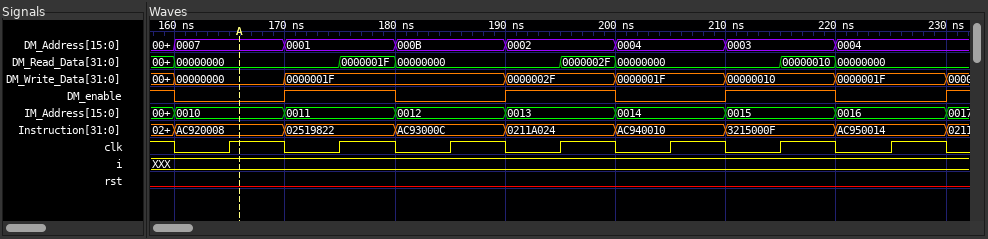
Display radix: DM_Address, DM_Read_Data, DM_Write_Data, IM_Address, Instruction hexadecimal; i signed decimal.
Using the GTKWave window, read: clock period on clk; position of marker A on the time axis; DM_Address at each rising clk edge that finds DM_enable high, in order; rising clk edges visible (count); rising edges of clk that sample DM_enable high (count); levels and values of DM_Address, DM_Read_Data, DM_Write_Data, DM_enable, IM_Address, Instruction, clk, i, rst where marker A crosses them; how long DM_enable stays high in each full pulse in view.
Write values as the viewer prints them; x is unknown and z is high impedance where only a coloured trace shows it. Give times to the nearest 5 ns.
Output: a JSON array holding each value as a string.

["10 ns", "165 ns", "0001, 0002, 0003", "7", "3", "DM_Address=0007, DM_Read_Data=00000000, DM_Write_Data=00000000, DM_enable=0, IM_Address=0010, Instruction=AC920008, clk=1, i=XXX, rst=0", "10 ns, 10 ns, 10 ns"]
